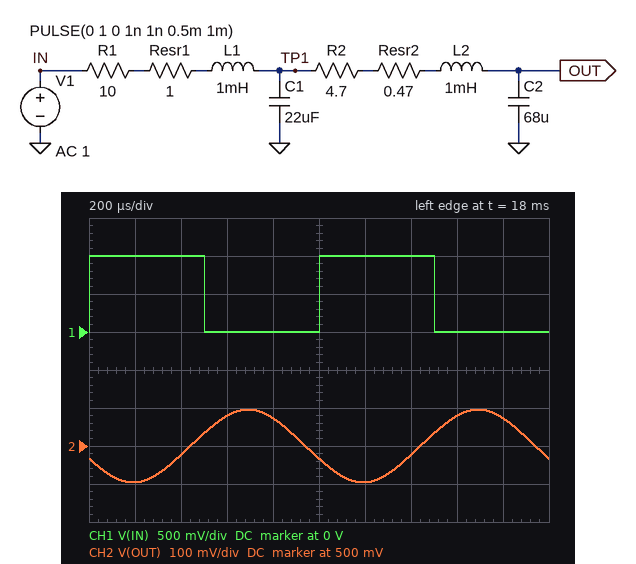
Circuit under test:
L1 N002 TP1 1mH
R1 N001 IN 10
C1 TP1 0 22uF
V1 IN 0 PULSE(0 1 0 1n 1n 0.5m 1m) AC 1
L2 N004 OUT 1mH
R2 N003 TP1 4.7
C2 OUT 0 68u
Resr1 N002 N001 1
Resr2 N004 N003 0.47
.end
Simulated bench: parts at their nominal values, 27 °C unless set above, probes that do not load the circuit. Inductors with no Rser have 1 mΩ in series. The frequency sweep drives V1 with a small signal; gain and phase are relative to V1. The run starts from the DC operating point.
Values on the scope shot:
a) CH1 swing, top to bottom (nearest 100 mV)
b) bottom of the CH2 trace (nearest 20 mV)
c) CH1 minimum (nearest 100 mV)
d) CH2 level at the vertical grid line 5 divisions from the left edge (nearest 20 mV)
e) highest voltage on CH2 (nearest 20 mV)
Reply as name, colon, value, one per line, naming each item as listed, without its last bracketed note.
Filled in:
CH1 swing, top to bottom: 1.0 V
bottom of the CH2 trace: 400 mV
CH1 minimum: 0 V
CH2 level at the vertical grid line 5 divisions from the left edge: 460 mV
highest voltage on CH2: 600 mV
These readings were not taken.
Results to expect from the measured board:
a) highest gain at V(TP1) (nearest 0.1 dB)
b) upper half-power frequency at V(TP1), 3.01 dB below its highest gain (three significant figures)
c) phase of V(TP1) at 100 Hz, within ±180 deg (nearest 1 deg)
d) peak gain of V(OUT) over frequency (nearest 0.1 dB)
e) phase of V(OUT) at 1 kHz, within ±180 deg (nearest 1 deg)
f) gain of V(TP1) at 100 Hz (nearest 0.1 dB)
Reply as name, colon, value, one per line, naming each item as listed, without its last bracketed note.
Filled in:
highest gain at V(TP1): 0 dB
upper half-power frequency at V(TP1), 3.01 dB below its highest gain: 138 Hz
phase of V(TP1) at 100 Hz, within ±180 deg: -30 deg
peak gain of V(OUT) over frequency: 0 dB
phase of V(OUT) at 1 kHz, within ±180 deg: -159 deg
gain of V(TP1) at 100 Hz: -1.8 dB
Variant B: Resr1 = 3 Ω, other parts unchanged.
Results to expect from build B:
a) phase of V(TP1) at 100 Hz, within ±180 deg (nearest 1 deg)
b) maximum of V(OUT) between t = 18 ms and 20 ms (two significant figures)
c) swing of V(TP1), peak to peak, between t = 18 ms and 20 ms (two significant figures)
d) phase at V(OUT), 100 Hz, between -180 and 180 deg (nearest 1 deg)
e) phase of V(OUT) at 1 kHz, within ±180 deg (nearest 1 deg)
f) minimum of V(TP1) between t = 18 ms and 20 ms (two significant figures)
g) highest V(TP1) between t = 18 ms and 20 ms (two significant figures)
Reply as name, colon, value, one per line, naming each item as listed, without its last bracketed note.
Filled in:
phase of V(TP1) at 100 Hz, within ±180 deg: -34 deg
maximum of V(OUT) between t = 18 ms and 20 ms: 590 mV
swing of V(TP1), peak to peak, between t = 18 ms and 20 ms: 460 mV
phase at V(OUT), 100 Hz, between -180 and 180 deg: -47 deg
phase of V(OUT) at 1 kHz, within ±180 deg: -158 deg
minimum of V(TP1) between t = 18 ms and 20 ms: 270 mV
highest V(TP1) between t = 18 ms and 20 ms: 730 mV
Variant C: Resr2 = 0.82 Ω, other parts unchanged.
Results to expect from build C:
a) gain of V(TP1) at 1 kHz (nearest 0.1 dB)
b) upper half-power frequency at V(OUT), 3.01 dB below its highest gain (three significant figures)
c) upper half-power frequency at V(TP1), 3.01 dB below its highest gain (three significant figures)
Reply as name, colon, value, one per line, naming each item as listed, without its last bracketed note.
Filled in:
gain of V(TP1) at 1 kHz: -7.6 dB
upper half-power frequency at V(OUT), 3.01 dB below its highest gain: 136 Hz
upper half-power frequency at V(TP1), 3.01 dB below its highest gain: 137 Hz
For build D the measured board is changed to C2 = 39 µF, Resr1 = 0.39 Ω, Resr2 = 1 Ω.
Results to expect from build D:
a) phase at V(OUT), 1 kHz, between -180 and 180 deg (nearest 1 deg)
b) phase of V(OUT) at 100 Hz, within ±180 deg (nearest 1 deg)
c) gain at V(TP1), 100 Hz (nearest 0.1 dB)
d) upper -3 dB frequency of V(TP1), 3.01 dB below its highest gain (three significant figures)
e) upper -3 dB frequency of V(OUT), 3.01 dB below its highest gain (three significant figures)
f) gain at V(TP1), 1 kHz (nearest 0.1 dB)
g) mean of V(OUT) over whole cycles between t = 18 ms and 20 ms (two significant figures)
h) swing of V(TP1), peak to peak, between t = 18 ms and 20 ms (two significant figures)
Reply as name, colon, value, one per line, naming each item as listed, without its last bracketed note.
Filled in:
phase at V(OUT), 1 kHz, between -180 and 180 deg: -152 deg
phase of V(OUT) at 100 Hz, within ±180 deg: -30 deg
gain at V(TP1), 100 Hz: -0.7 dB
upper -3 dB frequency of V(TP1), 3.01 dB below its highest gain: 229 Hz
upper -3 dB frequency of V(OUT), 3.01 dB below its highest gain: 242 Hz
gain at V(TP1), 1 kHz: -8.8 dB
mean of V(OUT) over whole cycles between t = 18 ms and 20 ms: 500 mV
swing of V(TP1), peak to peak, between t = 18 ms and 20 ms: 430 mV
